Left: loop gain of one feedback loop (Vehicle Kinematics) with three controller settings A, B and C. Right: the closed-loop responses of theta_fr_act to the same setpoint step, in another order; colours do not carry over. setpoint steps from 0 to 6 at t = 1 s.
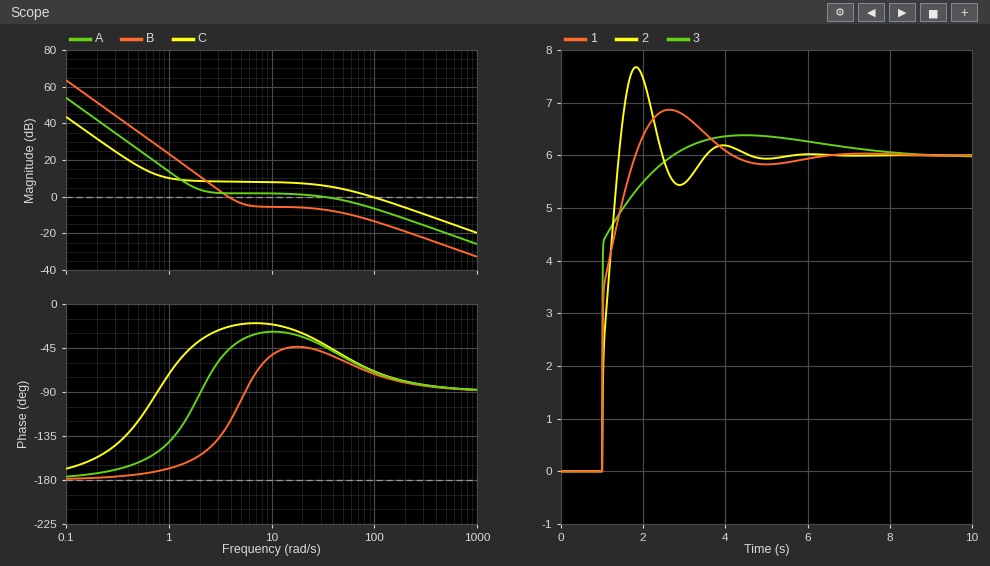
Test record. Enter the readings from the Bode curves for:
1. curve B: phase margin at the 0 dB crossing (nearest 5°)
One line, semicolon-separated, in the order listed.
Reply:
55°
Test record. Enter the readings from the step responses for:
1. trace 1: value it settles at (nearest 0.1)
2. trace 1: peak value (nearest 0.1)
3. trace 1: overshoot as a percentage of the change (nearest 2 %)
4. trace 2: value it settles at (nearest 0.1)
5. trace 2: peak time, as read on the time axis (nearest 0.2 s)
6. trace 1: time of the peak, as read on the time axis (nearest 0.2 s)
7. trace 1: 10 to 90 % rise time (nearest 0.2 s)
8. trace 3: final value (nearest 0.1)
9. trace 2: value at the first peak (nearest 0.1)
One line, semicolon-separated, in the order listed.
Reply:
6.0; 6.9; 14 %; 6.0; 1.8 s; 2.6 s; 0.6 s; 6.0; 7.7
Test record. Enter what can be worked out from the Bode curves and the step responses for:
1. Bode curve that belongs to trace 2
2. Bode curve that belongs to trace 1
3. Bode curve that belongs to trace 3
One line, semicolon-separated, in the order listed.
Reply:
B; A; C
